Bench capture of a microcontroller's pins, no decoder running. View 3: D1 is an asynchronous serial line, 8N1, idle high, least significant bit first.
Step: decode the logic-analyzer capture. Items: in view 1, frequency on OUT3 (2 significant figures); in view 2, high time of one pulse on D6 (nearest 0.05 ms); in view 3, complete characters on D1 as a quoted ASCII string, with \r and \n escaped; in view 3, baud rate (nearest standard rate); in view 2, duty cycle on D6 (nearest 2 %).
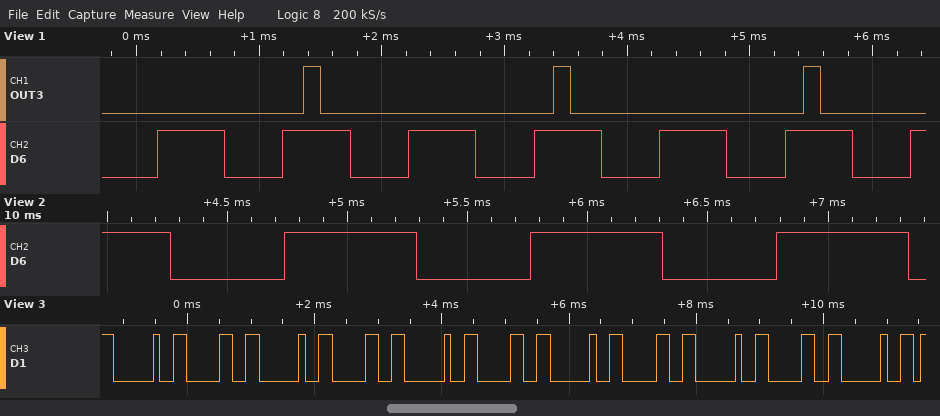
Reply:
490 Hz
0.55 ms
" 0 0 0 0 0 "
9600 baud
54 %
